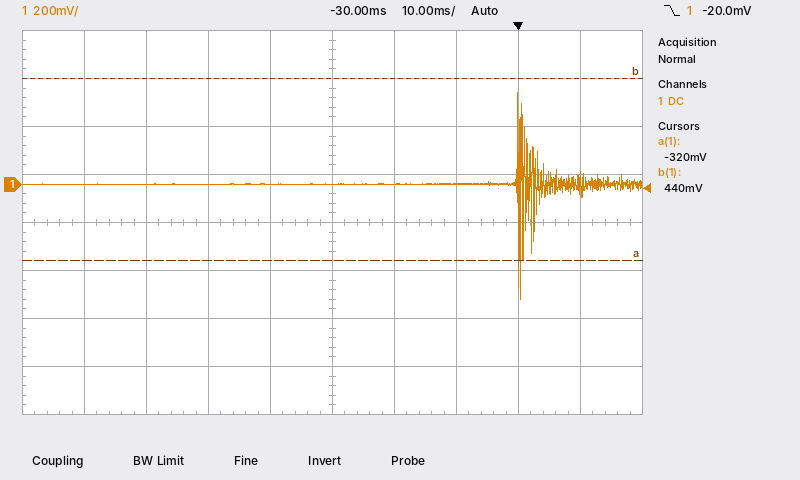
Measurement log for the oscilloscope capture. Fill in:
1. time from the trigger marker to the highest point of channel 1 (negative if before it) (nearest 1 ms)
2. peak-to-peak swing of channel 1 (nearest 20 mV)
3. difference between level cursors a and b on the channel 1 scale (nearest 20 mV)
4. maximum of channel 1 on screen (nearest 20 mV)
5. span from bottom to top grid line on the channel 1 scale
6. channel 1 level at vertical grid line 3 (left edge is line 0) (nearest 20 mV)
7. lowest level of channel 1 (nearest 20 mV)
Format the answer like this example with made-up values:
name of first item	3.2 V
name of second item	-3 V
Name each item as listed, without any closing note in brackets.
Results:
time from the trigger marker to the highest point of channel 1 (negative if before it)	0 ms
peak-to-peak swing of channel 1	860 mV
difference between level cursors a and b on the channel 1 scale	760 mV
maximum of channel 1 on screen	380 mV
span from bottom to top grid line on the channel 1 scale	1.6 V
channel 1 level at vertical grid line 3 (left edge is line 0)	0 mV
lowest level of channel 1	-480 mV
